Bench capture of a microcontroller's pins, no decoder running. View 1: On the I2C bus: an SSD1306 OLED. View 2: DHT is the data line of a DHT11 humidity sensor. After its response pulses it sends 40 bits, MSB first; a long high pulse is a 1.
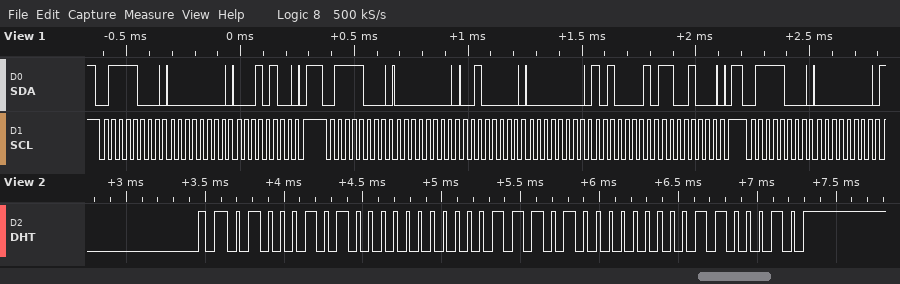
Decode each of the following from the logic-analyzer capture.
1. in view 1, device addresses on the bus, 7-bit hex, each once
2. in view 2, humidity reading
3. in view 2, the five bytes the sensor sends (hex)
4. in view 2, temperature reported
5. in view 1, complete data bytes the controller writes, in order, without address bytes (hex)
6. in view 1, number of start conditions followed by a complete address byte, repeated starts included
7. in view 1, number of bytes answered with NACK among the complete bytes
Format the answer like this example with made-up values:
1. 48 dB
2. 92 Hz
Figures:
1. 0x3C
2. 69 %
3. 45 00 1D 00 62
4. 29.0 °C
5. 00 14 00 20 00 A1 C8 00
6. 3
7. 0
